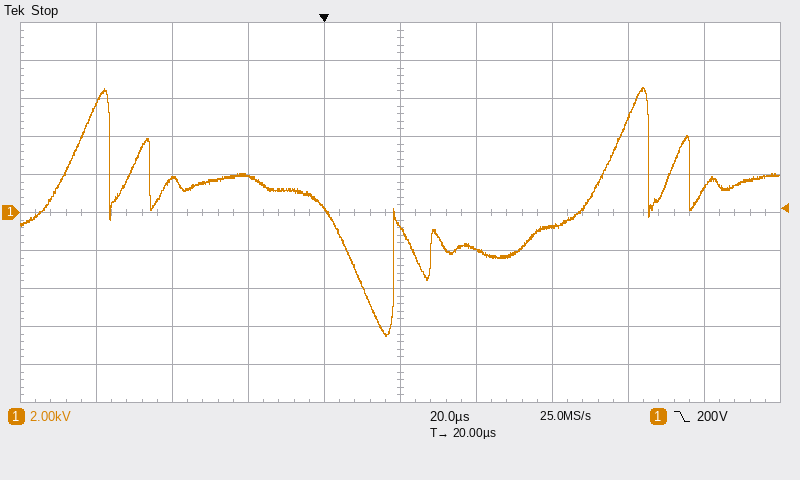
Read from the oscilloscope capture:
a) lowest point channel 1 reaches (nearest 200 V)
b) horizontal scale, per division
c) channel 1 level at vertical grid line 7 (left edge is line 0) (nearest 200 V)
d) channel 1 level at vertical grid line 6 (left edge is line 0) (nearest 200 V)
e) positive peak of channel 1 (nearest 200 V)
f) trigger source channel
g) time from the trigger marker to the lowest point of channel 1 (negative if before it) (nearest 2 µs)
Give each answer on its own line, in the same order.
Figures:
-6.6 kV
20 µs
-800 V
-2.0 kV
6.6 kV
channel 1
+16 µs
